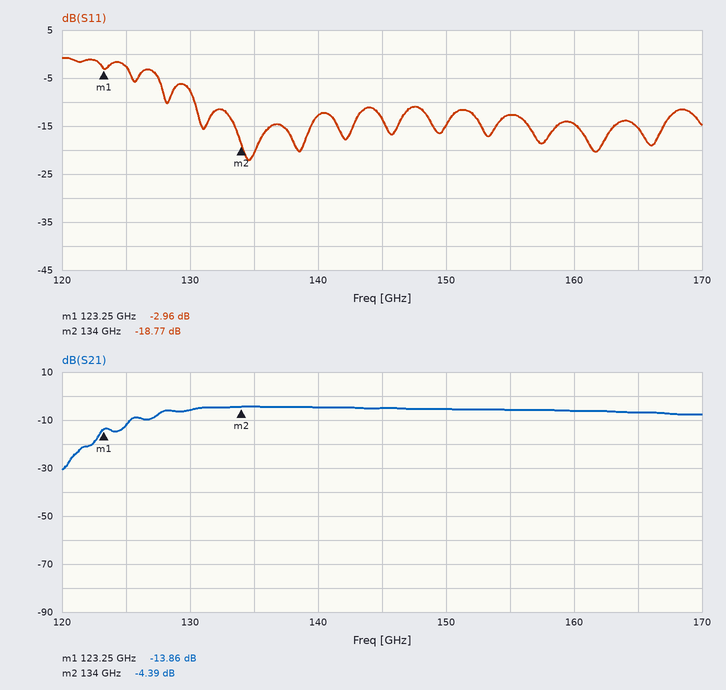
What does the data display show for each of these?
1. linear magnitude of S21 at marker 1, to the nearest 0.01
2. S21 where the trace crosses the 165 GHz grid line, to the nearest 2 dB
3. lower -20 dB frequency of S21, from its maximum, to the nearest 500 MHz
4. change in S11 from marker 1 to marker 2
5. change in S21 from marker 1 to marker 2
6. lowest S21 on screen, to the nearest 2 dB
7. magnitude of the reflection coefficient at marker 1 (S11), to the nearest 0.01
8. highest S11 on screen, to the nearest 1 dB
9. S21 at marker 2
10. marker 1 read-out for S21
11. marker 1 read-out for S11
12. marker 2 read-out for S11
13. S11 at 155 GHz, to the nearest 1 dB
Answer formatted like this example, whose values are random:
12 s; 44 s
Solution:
0.20; -6 dB; 121.0 GHz; -15.81 dB; 9.47 dB; -30 dB; 0.71; -1 dB; -4.39 dB; -13.86 dB; -2.96 dB; -18.77 dB; -13 dB
